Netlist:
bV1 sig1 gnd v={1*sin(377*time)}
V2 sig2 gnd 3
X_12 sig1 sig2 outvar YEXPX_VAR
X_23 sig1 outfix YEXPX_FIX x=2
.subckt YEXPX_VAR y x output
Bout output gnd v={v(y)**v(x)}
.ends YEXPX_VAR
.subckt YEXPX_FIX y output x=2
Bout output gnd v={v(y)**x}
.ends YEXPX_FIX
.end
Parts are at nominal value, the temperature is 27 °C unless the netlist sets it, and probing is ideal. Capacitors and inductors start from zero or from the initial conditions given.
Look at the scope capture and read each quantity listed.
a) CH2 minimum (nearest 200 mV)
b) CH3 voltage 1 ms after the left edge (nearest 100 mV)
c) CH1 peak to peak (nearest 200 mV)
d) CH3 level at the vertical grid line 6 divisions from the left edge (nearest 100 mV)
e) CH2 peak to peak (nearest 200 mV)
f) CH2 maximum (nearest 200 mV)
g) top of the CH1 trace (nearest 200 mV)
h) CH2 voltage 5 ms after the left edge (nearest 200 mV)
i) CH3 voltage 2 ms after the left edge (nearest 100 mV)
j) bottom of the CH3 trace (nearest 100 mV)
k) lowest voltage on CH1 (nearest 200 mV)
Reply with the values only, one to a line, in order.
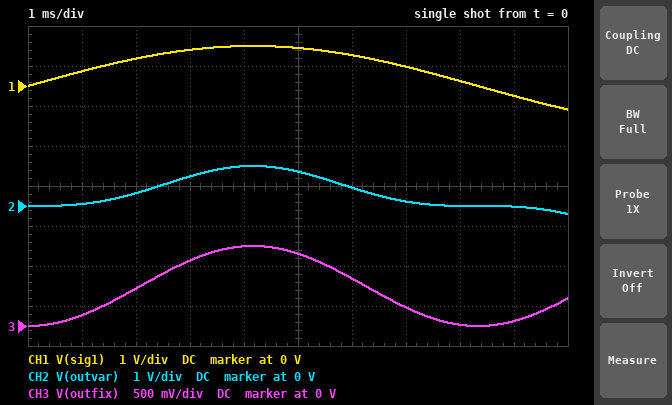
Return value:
-200 mV
100 mV
1.6 V
600 mV
1.2 V
1.0 V
1.0 V
800 mV
500 mV
0 V
-600 mV
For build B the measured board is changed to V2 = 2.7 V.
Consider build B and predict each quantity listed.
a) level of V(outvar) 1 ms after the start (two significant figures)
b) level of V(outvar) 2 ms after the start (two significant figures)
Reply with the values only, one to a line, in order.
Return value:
67 mV
360 mV
